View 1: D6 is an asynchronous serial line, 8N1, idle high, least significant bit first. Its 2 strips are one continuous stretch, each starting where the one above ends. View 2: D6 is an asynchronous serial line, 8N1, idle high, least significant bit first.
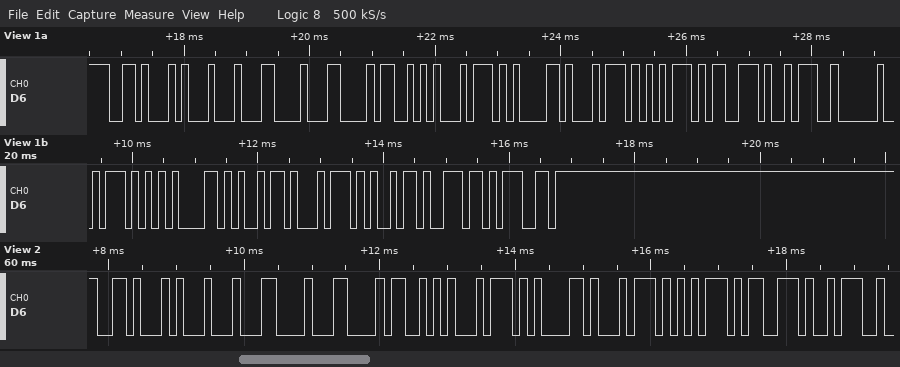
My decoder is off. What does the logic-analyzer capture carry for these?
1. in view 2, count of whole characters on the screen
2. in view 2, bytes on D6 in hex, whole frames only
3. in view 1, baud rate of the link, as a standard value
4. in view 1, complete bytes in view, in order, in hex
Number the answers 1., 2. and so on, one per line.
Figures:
1. 11
2. 16 11 0C 0C 53 74 61 74 75 73 3A
3. 9600 baud
4. 0x16 0x11 0x0C 0x0C 0x53 0x74 0x61 0x74 0x75 0x73 0x3A 0x20 0x57 0x61 0x69 0x74 0x69 0x6E 0x67
